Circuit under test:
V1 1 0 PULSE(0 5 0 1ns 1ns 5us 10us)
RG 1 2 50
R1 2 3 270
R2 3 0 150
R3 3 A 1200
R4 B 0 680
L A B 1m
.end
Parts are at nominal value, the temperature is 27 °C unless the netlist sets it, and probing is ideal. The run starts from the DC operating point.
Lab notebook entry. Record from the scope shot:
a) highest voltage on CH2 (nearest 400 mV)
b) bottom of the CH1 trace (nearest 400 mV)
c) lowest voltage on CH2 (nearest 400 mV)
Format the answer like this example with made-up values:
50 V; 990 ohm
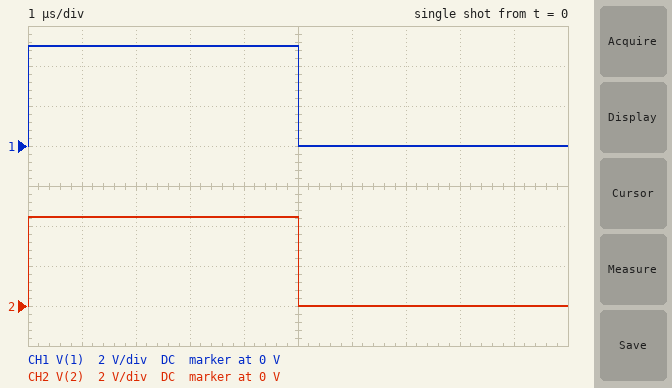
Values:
4.4 V; 0 V; 0 V
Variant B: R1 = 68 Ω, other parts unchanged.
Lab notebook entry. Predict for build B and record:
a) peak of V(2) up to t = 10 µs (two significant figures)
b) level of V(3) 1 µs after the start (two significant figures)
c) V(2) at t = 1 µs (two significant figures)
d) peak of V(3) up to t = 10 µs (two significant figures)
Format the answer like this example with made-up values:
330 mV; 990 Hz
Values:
4.1 V; 2.7 V; 4.0 V; 2.8 V
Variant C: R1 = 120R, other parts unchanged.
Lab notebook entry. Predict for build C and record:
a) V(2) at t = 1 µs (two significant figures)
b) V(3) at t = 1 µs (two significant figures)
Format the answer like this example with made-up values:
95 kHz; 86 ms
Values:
4.2 V; 2.3 V
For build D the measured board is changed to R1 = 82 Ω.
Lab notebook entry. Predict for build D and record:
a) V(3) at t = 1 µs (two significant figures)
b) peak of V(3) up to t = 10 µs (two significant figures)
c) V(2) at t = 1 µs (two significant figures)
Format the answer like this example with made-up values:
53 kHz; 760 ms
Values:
2.6 V; 2.7 V; 4.1 V
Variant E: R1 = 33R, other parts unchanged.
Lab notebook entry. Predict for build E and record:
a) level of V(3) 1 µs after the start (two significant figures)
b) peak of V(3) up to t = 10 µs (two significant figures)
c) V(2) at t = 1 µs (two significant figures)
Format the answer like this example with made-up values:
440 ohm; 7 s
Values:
3.1 V; 3.2 V; 3.9 V
